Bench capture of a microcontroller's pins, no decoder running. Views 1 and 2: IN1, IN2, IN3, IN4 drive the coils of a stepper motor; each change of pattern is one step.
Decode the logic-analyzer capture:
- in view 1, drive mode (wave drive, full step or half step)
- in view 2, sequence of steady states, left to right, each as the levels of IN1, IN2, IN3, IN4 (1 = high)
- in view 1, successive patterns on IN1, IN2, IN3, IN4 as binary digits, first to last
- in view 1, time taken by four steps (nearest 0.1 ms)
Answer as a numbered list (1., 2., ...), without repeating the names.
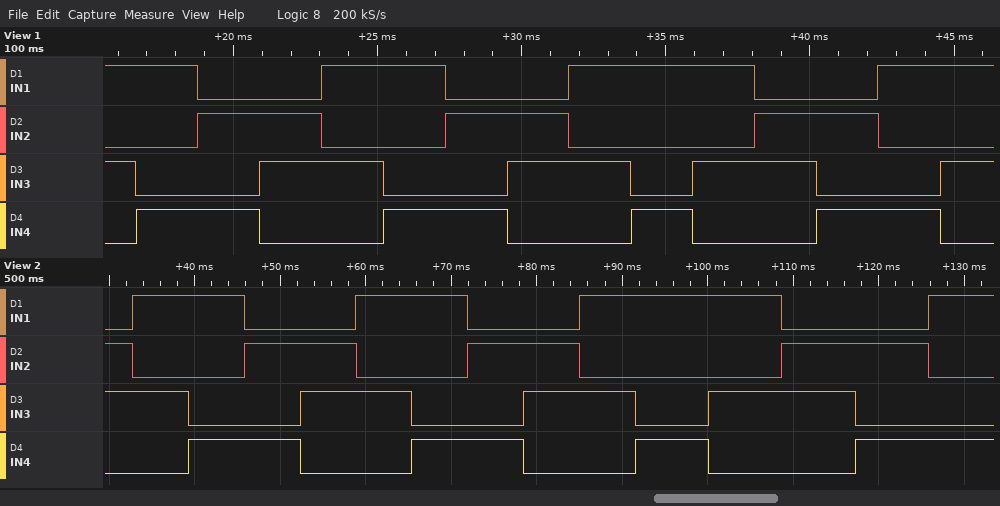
1. full step
2. 0110 1010 1001 0101 0110 1010 1001 0101 0110 1010 1001 1010 0110 0101 1001
3. 1010 1001 0101 0110 1010 1001 0101 0110 1010 1001 1010 0110 0101 1001 1010
4. 8.6 ms
